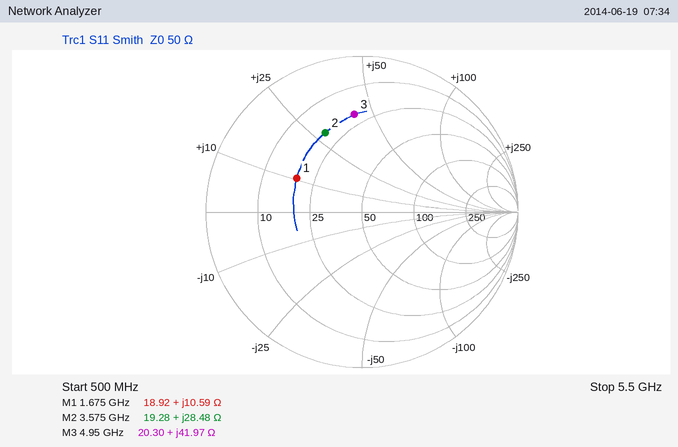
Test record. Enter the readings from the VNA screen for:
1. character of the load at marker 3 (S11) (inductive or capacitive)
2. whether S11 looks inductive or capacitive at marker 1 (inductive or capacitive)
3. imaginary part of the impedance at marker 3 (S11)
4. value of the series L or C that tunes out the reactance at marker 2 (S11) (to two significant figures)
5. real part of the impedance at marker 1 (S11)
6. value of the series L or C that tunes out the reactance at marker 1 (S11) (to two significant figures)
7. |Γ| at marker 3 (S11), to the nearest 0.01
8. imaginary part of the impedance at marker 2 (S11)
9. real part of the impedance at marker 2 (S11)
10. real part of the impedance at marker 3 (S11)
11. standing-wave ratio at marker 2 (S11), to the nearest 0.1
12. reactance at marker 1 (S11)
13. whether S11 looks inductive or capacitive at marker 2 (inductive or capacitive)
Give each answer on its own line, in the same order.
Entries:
inductive
inductive
+41.97 Ω
1.6 pF
18.92 Ω
9.0 pF
0.63
+28.48 Ω
19.28 Ω
20.30 Ω
3.5
+10.59 Ω
inductive
